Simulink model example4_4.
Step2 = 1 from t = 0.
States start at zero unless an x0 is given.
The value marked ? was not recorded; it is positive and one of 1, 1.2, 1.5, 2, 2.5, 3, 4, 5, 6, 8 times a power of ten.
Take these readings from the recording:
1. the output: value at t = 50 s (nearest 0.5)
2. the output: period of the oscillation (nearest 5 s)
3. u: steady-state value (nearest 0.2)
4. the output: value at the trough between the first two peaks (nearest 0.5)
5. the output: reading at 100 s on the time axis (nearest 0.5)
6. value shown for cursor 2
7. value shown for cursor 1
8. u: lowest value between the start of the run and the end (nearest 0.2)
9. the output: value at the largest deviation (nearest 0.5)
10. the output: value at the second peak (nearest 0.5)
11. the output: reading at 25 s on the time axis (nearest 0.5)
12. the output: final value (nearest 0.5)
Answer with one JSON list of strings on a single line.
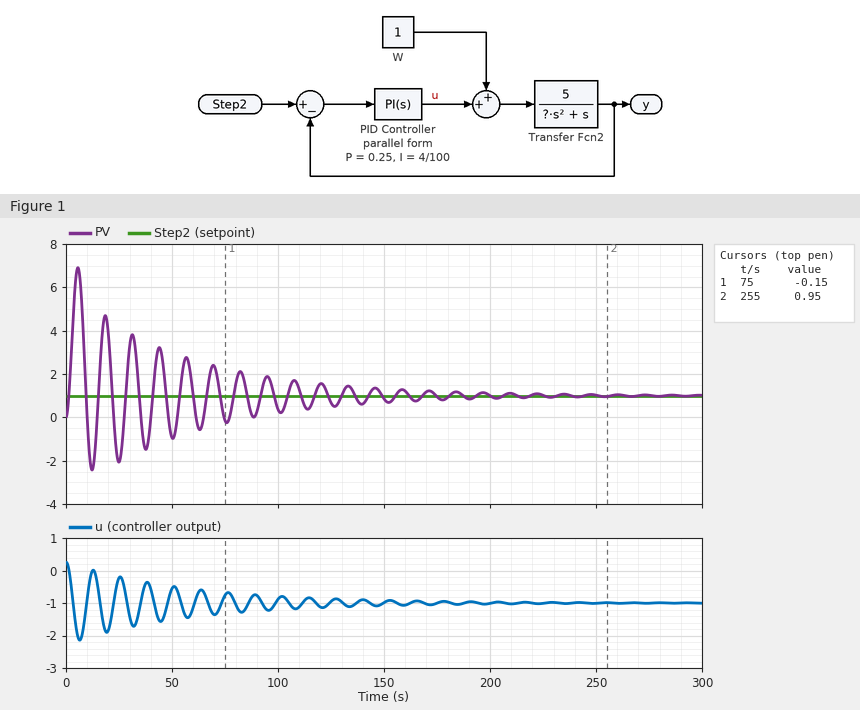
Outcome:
["-1.0", "15 s", "-1.0", "-2.5", "0.5", "0.95", "-0.15", "-2.2", "7.0", "4.5", "-2.0", "1.0"]
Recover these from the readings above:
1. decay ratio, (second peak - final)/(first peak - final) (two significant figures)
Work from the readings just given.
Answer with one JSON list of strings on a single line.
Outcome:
["0.58"]
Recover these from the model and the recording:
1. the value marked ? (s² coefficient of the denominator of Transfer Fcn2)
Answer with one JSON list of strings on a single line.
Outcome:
["5"]
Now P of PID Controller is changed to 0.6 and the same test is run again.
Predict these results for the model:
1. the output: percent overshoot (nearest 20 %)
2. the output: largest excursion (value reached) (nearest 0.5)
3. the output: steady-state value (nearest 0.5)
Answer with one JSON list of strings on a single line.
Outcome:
["340 %", "4.5", "1.0"]
